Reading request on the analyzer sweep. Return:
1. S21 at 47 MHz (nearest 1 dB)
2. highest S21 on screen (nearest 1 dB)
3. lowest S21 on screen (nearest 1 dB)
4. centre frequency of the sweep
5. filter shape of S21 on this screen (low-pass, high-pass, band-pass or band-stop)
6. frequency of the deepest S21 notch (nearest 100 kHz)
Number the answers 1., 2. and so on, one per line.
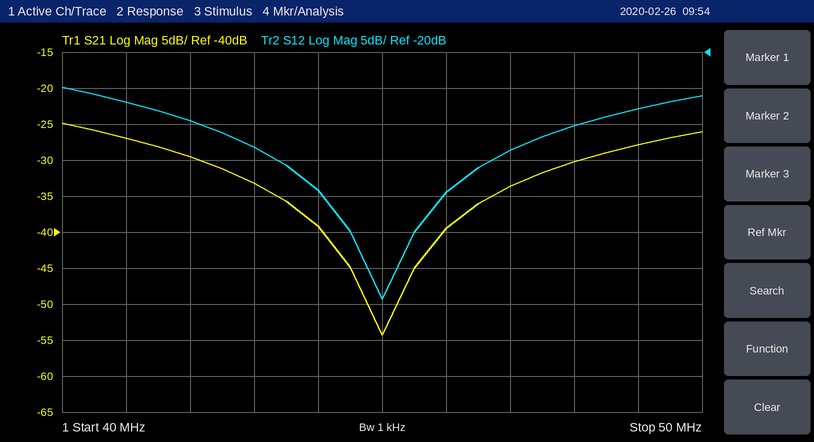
1. -34 dB
2. -25 dB
3. -54 dB
4. 45 MHz
5. band-stop
6. 45.0 MHz
